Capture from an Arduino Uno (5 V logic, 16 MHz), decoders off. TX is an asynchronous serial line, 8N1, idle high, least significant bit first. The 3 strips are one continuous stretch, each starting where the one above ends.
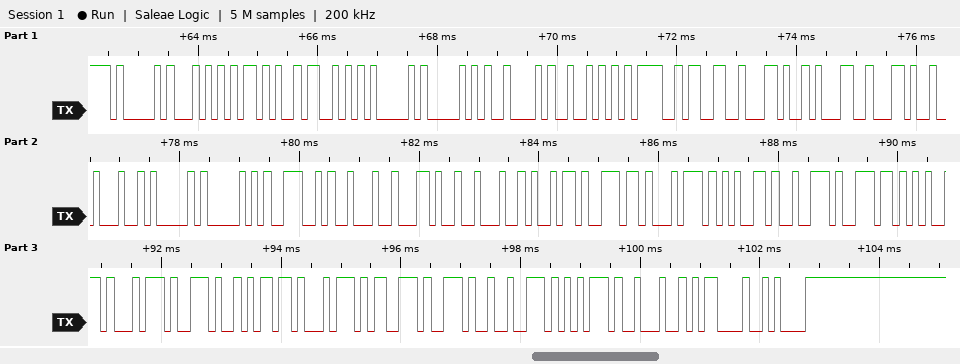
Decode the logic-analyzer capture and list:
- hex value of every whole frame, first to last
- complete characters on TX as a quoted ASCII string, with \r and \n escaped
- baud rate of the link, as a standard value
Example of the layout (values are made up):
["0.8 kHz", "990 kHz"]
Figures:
["0x41 0x54 0x2B 0x53 0x41 0x50 0x42 0x52 0x3D 0x33 0x2C 0x31 0x2C 0x22 0x41 0x50 0x4E 0x22 0x2C 0x22 0x69 0x6E 0x74 0x65 0x72 0x6E 0x65 0x74 0x2E 0x6D 0x74 0x73 0x2E 0x72 0x75 0x22 0x0D 0x0A", "\"AT+SAPBR=3,1,\\\"APN\\\",\\\"internet.mts.ru\\\"\\r\\n\"", "9600 baud"]
